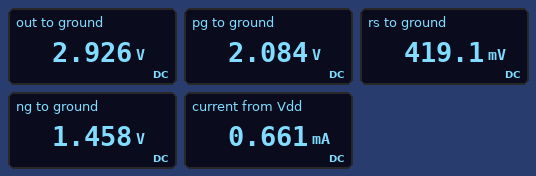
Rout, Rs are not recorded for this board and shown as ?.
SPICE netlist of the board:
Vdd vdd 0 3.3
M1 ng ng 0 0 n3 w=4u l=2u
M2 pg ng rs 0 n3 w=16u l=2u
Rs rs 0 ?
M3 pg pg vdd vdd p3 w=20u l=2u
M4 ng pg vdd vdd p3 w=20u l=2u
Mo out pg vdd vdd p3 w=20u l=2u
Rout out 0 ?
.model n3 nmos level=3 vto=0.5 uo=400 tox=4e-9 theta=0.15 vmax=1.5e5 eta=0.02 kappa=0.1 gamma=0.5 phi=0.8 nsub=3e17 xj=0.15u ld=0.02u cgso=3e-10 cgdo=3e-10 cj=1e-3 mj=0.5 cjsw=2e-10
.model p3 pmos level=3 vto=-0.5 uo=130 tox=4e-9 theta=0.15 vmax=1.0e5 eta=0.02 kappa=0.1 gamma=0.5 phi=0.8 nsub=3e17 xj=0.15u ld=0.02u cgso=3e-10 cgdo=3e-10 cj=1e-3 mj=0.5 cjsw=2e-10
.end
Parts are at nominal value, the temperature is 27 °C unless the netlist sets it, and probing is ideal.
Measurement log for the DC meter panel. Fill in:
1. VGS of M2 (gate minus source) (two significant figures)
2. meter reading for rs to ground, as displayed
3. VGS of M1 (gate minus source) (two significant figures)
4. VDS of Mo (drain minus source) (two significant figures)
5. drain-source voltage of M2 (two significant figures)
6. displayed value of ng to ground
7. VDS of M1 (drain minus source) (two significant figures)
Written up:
1.0 V
419.1 mV
1.5 V
-370 mV
1.7 V
1.458 V
1.5 V
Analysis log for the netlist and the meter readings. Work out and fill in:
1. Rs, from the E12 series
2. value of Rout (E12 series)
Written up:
1.8 kΩ
15 kΩ
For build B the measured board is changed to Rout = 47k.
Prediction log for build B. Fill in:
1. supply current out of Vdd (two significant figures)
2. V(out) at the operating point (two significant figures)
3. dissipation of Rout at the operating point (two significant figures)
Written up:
530 µA
3.2 V
220 µW
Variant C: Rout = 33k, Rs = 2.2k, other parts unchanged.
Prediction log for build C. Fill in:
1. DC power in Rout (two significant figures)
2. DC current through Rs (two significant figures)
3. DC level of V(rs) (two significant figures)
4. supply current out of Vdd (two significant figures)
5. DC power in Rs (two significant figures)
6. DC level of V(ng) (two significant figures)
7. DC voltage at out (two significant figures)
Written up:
290 µW
140 µA
320 mV
380 µA
46 µW
1.2 V
3.1 V
